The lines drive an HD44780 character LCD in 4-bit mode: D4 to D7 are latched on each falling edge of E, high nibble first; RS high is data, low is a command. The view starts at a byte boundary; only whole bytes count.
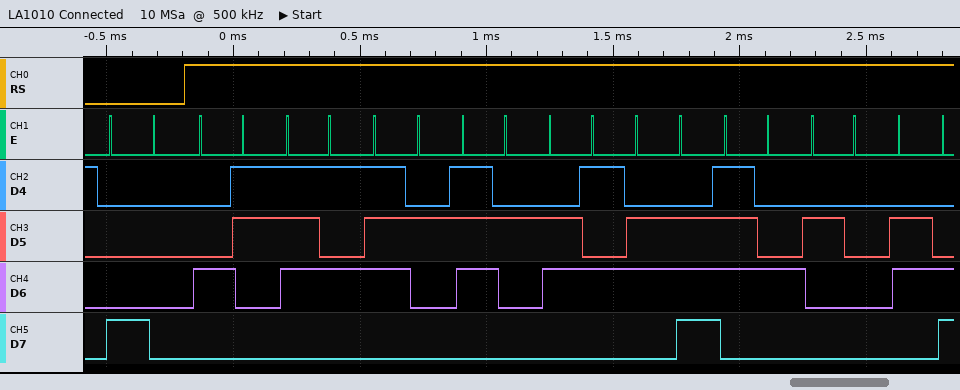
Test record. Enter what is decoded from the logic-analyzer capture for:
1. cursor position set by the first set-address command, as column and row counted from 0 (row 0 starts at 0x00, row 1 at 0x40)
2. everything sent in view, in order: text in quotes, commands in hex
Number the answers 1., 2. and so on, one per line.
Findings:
1. column 0, row 0
2. 0x80 "Current l"
